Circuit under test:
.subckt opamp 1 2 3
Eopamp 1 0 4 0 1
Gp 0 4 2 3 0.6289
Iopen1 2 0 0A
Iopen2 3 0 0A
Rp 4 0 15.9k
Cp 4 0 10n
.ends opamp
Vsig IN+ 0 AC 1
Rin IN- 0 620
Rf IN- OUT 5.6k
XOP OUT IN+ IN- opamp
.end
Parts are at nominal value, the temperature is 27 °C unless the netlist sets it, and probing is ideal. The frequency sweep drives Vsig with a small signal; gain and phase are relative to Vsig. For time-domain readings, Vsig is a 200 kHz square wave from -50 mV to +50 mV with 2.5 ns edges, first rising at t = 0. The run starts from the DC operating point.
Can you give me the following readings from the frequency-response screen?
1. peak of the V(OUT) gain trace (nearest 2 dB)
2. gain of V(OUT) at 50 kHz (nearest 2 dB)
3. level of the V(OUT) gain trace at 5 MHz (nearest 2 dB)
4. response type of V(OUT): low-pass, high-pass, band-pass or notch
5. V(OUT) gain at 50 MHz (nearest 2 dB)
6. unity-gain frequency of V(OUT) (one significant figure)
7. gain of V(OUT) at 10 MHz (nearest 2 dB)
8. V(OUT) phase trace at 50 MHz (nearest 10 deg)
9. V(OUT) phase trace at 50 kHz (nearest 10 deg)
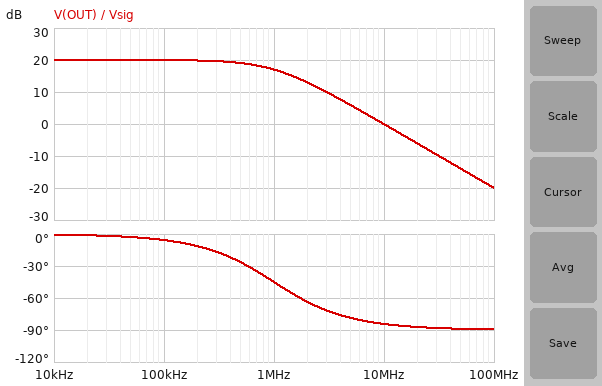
20 dB
20 dB
6 dB
low-pass
-14 dB
10 MHz
0 dB
-90 deg
0 deg
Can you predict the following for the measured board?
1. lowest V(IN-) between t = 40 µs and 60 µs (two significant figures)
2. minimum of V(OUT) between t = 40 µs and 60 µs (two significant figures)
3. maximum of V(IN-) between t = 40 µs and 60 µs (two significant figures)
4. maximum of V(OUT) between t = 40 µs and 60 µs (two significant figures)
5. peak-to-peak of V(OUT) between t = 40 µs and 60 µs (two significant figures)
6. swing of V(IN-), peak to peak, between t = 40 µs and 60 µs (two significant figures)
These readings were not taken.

-50 mV
-500 mV
50 mV
500 mV
1.0 V
100 mV
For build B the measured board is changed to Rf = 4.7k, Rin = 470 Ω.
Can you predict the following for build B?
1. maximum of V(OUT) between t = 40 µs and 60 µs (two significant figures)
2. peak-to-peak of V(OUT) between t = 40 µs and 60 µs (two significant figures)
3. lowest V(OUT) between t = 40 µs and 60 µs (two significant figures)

550 mV
1.1 V
-550 mV
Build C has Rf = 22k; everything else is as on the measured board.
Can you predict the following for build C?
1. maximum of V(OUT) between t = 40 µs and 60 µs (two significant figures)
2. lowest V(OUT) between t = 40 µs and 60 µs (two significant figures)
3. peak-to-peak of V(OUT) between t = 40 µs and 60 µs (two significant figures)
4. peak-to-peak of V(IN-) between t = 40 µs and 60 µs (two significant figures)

1.8 V
-1.8 V
3.5 V
97 mV
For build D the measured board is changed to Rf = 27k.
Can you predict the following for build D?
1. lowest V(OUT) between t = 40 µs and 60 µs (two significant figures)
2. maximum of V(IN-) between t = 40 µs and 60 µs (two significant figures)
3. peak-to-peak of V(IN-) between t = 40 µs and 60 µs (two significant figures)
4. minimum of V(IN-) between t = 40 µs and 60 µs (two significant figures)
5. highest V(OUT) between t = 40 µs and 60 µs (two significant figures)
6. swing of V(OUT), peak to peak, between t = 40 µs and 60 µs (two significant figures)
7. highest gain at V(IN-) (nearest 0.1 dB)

-2.1 V
47 mV
94 mV
-47 mV
2.1 V
4.2 V
0 dB
